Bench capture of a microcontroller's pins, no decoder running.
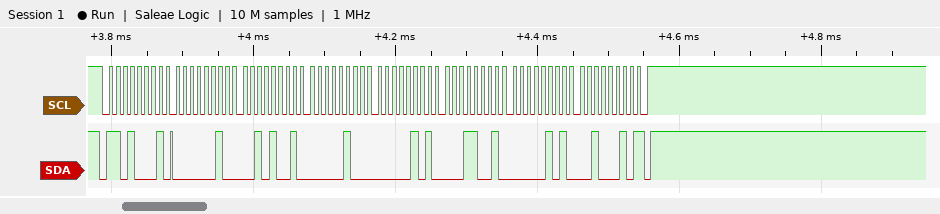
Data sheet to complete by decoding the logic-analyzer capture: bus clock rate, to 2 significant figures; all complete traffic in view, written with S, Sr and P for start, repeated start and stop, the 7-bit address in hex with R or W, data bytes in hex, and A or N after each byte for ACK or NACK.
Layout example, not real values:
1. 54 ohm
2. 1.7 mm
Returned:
1. 100 kHz
2. S 68R A 02 A 29 A 04 A 05 A 19 A 05 A 22 N P
